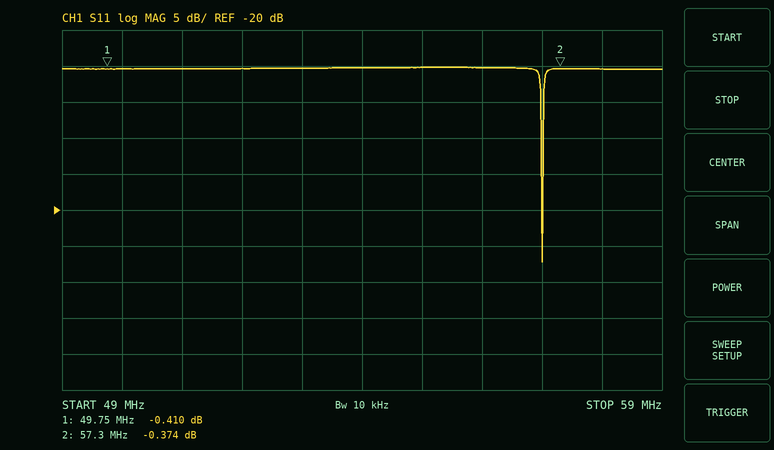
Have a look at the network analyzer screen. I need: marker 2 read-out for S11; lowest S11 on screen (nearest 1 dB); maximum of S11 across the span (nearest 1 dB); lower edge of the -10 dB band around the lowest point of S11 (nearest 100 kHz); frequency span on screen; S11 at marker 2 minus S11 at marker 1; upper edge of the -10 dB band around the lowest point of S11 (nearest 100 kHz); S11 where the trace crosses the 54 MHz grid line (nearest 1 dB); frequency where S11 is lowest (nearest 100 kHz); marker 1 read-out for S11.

-0.374 dB
-27 dB
0 dB
57.0 MHz
10 MHz
0.036 dB
57.0 MHz
0 dB
57.0 MHz
-0.410 dB
